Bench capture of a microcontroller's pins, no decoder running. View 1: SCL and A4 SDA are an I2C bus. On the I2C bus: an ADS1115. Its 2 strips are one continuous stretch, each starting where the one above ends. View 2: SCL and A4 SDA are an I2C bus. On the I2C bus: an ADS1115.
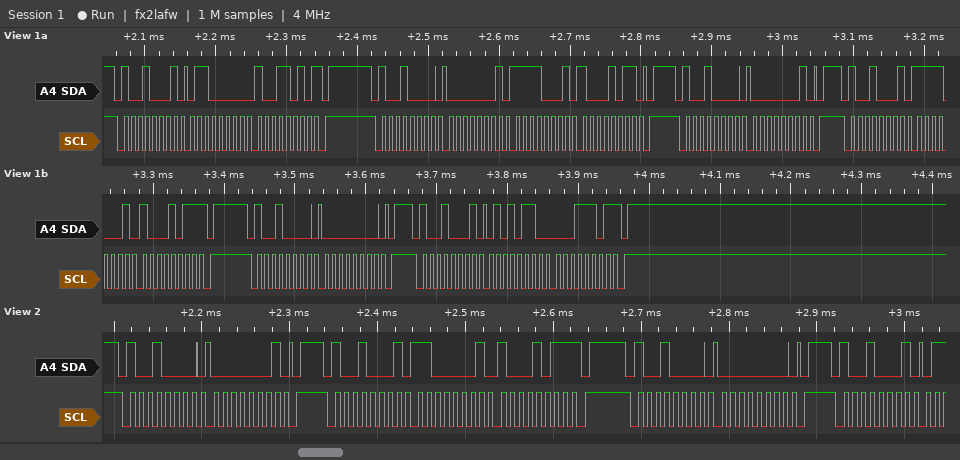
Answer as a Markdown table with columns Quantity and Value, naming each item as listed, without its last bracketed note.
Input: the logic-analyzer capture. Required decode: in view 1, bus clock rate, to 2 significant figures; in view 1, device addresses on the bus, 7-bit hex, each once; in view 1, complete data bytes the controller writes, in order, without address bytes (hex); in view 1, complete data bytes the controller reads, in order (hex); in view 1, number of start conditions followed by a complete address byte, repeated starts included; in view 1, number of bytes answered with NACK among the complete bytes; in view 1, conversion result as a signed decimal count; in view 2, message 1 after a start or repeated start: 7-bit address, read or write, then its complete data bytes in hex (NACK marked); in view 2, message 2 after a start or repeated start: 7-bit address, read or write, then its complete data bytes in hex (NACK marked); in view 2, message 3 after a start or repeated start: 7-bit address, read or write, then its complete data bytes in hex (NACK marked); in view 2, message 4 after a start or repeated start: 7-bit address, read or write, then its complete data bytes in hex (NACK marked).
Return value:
| Quantity | Value |
|---|---|
| in view 1, bus clock rate, to 2 significant figures | 100 kHz |
| in view 1, device addresses on the bus, 7-bit hex, each once | 0x48 |
| in view 1, complete data bytes the controller writes, in order, without address bytes | 01 F1 8B 01 00 |
| in view 1, complete data bytes the controller reads, in order | 60 9A F1 8B 56 1D |
| in view 1, number of start conditions followed by a complete address byte, repeated starts included | 6 |
| in view 1, number of bytes answered with NACK among the complete bytes | 3 |
| in view 1, conversion result as a signed decimal count | 22045 |
| in view 2, message 1 after a start or repeated start: 7-bit address, read or write, then its complete data bytes in hex | 0x48 write: 01 |
| in view 2, message 2 after a start or repeated start: 7-bit address, read or write, then its complete data bytes in hex | 0x48 read: C1 8B NACK |
| in view 2, message 3 after a start or repeated start: 7-bit address, read or write, then its complete data bytes in hex | 0x48 write: 00 |
| in view 2, message 4 after a start or repeated start: 7-bit address, read or write, then its complete data bytes in hex | 0x48 read |
